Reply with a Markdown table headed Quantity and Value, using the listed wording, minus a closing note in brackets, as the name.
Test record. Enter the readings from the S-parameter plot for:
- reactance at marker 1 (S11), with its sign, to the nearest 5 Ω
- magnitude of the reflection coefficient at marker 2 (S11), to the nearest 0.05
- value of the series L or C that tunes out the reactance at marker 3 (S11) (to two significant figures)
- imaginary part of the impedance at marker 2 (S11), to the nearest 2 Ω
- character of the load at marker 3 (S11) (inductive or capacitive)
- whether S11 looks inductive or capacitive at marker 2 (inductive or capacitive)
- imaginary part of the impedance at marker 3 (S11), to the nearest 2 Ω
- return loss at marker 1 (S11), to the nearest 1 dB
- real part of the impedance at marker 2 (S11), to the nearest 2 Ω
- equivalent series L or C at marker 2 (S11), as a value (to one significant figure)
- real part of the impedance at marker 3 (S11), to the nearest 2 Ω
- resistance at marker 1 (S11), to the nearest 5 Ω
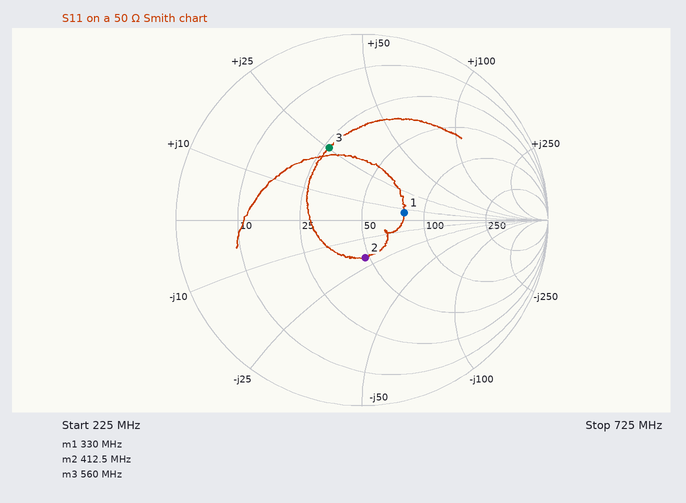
| Quantity | Value |
|---|---|
| reactance at marker 1 (S11), with its sign, to the nearest 5 Ω | +5 Ω |
| magnitude of the reflection coefficient at marker 2 (S11), to the nearest 0.05 | 0.20 |
| value of the series L or C that tunes out the reactance at marker 3 (S11) | 11 pF |
| imaginary part of the impedance at marker 2 (S11), to the nearest 2 Ω | -20 Ω |
| character of the load at marker 3 (S11) | inductive |
| whether S11 looks inductive or capacitive at marker 2 | capacitive |
| imaginary part of the impedance at marker 3 (S11), to the nearest 2 Ω | +26 Ω |
| return loss at marker 1 (S11), to the nearest 1 dB | 13 dB |
| real part of the impedance at marker 2 (S11), to the nearest 2 Ω | 48 Ω |
| equivalent series L or C at marker 2 (S11), as a value | 20 pF |
| real part of the impedance at marker 3 (S11), to the nearest 2 Ω | 26 Ω |
| resistance at marker 1 (S11), to the nearest 5 Ω | 80 Ω |
